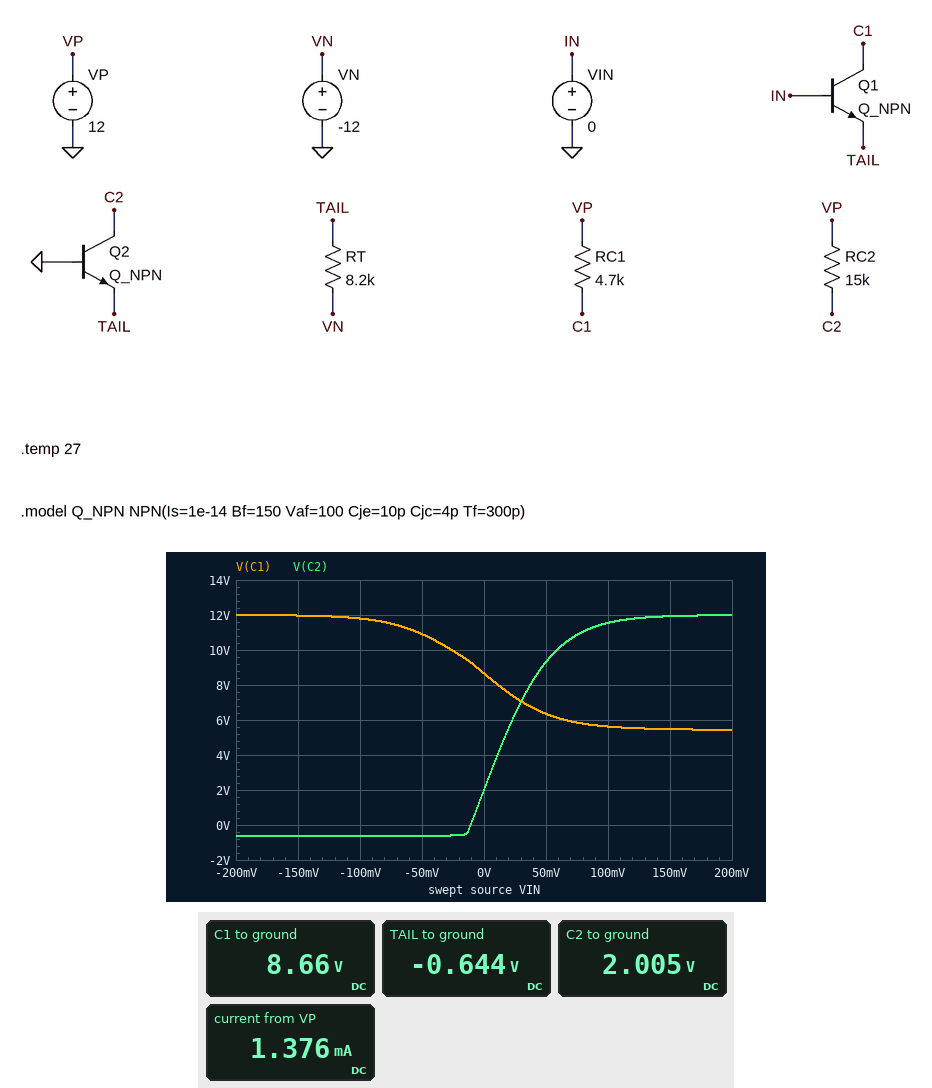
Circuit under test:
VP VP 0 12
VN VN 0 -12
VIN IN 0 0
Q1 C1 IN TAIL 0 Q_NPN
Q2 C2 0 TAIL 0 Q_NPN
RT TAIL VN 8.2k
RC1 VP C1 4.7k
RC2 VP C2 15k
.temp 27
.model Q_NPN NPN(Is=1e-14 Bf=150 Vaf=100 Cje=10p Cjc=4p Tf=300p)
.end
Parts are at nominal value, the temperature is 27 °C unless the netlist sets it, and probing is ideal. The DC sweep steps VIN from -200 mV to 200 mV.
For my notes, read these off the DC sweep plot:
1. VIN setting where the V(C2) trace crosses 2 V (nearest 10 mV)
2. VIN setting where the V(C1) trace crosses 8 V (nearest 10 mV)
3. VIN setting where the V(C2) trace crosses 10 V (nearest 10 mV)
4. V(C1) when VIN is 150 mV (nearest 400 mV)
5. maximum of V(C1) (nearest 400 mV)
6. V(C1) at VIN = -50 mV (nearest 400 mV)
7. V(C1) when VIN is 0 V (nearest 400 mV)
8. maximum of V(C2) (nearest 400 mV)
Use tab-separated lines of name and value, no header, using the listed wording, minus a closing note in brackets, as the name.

VIN setting where the V(C2) trace crosses 2 V	0 V
VIN setting where the V(C1) trace crosses 8 V	10 mV
VIN setting where the V(C2) trace crosses 10 V	60 mV
V(C1) when VIN is 150 mV	5.6 V
maximum of V(C1)	12.0 V
V(C1) at VIN = -50 mV	10.8 V
V(C1) when VIN is 0 V	8.8 V
maximum of V(C2)	12.0 V
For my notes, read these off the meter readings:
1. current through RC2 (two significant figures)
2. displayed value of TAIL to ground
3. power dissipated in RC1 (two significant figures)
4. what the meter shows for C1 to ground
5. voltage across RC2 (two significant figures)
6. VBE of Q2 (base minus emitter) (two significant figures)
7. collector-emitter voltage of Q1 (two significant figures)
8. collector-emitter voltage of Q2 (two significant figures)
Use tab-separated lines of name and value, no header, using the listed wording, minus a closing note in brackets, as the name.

current through RC2	670 µA
displayed value of TAIL to ground	-0.644 V
power dissipated in RC1	2.4 mW
what the meter shows for C1 to ground	8.66 V
voltage across RC2	10 V
VBE of Q2 (base minus emitter)	640 mV
collector-emitter voltage of Q1	9.3 V
collector-emitter voltage of Q2	2.6 V
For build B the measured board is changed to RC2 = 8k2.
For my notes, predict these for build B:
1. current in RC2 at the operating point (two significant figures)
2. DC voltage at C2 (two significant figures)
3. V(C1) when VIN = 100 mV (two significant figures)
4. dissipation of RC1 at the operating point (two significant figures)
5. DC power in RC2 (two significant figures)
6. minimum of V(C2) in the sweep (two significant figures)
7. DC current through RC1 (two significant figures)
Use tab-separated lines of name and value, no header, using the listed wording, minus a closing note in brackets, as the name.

current in RC2 at the operating point	680 µA
DC voltage at C2	6.4 V
V(C1) when VIN = 100 mV	5.6 V
dissipation of RC1 at the operating point	2.3 mW
DC power in RC2	3.8 mW
minimum of V(C2) in the sweep	740 mV
DC current through RC1	700 µA
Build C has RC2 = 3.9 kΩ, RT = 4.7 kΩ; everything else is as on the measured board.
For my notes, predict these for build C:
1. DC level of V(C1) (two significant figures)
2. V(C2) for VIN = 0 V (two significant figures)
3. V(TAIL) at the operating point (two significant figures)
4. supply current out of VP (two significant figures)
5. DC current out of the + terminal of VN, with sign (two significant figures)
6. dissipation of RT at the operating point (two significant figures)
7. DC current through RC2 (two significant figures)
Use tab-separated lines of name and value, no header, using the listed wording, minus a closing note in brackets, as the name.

DC level of V(C1)	6.4 V
V(C2) for VIN = 0 V	7.3 V
V(TAIL) at the operating point	-660 mV
supply current out of VP	2.4 mA
DC current out of the + terminal of VN, with sign	-2.4 mA
dissipation of RT at the operating point	27 mW
DC current through RC2	1.2 mA
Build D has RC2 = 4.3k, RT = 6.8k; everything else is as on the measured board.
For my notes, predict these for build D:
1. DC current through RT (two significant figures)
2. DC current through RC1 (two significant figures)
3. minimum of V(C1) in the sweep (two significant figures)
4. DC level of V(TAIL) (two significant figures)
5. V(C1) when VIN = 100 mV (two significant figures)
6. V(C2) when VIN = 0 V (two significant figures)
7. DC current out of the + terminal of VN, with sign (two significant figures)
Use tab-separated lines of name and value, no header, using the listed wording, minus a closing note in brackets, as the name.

DC current through RT	1.7 mA
DC current through RC1	830 µA
minimum of V(C1) in the sweep	4.1 V
DC level of V(TAIL)	-650 mV
V(C1) when VIN = 100 mV	4.3 V
V(C2) when VIN = 0 V	8.4 V
DC current out of the + terminal of VN, with sign	-1.7 mA
